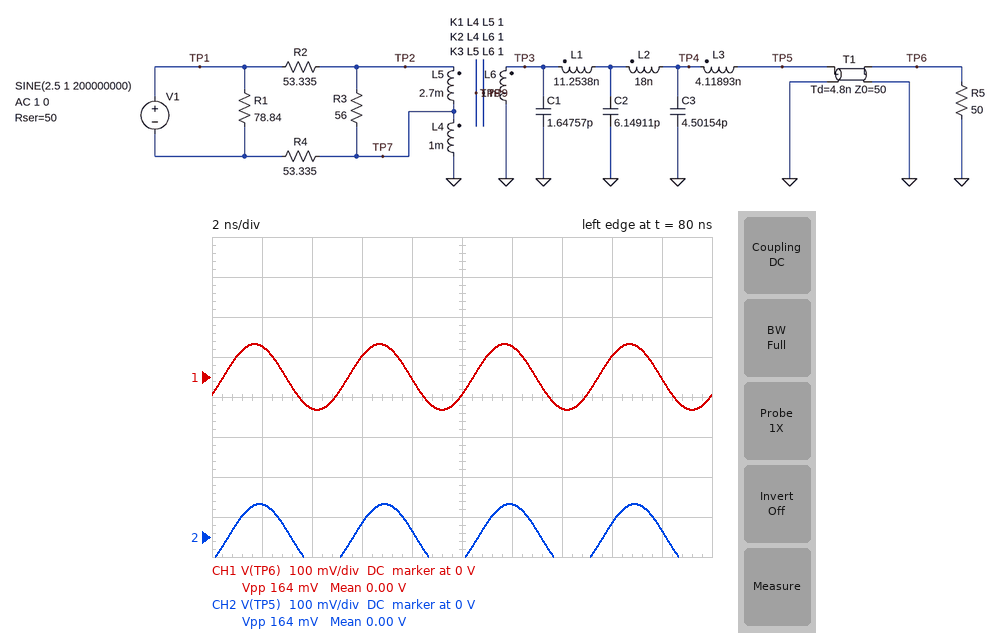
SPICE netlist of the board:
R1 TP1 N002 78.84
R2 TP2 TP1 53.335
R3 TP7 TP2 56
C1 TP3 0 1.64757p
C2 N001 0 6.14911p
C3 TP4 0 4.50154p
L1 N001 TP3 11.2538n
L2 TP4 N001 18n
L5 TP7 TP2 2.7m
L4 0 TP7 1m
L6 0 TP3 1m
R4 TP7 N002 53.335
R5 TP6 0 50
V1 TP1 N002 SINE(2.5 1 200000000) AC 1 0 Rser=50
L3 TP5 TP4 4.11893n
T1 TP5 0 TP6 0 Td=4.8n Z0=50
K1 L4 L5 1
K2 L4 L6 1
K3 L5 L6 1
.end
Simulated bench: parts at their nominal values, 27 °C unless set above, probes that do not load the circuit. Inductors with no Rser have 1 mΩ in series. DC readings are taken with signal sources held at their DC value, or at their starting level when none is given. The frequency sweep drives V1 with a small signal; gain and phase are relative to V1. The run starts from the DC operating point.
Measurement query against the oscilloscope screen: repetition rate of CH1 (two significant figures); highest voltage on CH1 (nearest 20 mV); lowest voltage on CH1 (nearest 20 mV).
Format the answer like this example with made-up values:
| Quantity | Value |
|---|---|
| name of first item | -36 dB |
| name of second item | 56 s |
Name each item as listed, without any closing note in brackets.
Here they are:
| Quantity | Value |
|---|---|
| repetition rate of CH1 | 200 MHz |
| highest voltage on CH1 | 80 mV |
| lowest voltage on CH1 | -80 mV |
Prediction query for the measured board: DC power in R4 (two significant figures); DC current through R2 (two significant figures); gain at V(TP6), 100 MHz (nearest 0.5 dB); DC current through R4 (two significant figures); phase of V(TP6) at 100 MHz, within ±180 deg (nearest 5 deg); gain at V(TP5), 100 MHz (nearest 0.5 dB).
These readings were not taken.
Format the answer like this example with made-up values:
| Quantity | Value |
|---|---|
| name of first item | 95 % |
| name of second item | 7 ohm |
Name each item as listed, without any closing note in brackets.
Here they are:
| Quantity | Value |
|---|---|
| DC power in R4 | 6.6 mW |
| DC current through R2 | 11 mA |
| gain at V(TP6), 100 MHz | -21.5 dB |
| DC current through R4 | 11 mA |
| phase of V(TP6) at 100 MHz, within ±180 deg | 165 deg |
| gain at V(TP5), 100 MHz | -21.5 dB |
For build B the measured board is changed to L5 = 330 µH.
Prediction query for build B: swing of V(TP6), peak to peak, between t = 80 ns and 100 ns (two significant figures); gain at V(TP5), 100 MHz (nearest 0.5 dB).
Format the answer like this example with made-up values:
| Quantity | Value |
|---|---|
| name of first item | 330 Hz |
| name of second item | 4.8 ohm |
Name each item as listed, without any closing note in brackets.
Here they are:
| Quantity | Value |
|---|---|
| swing of V(TP6), peak to peak, between t = 80 ns and 100 ns | 180 mV |
| gain at V(TP5), 100 MHz | -21.0 dB |
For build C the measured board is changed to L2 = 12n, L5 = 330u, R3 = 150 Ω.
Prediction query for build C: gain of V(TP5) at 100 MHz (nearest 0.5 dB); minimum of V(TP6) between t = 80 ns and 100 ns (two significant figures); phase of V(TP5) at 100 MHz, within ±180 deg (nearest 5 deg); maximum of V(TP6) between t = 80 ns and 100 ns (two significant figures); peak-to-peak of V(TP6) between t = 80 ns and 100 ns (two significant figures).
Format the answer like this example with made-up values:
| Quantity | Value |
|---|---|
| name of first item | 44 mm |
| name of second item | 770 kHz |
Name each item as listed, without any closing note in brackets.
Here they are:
| Quantity | Value |
|---|---|
| gain of V(TP5) at 100 MHz | -19.5 dB |
| minimum of V(TP6) between t = 80 ns and 100 ns | -100 mV |
| phase of V(TP5) at 100 MHz, within ±180 deg | -20 deg |
| maximum of V(TP6) between t = 80 ns and 100 ns | 100 mV |
| peak-to-peak of V(TP6) between t = 80 ns and 100 ns | 200 mV |
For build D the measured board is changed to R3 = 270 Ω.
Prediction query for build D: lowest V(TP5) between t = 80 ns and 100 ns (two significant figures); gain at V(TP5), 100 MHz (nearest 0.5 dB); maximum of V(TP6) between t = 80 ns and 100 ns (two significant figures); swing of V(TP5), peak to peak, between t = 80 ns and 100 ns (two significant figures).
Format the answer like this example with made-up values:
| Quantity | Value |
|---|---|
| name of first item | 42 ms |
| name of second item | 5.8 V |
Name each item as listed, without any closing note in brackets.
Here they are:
| Quantity | Value |
|---|---|
| lowest V(TP5) between t = 80 ns and 100 ns | -150 mV |
| gain at V(TP5), 100 MHz | -16.5 dB |
| maximum of V(TP6) between t = 80 ns and 100 ns | 150 mV |
| swing of V(TP5), peak to peak, between t = 80 ns and 100 ns | 290 mV |
